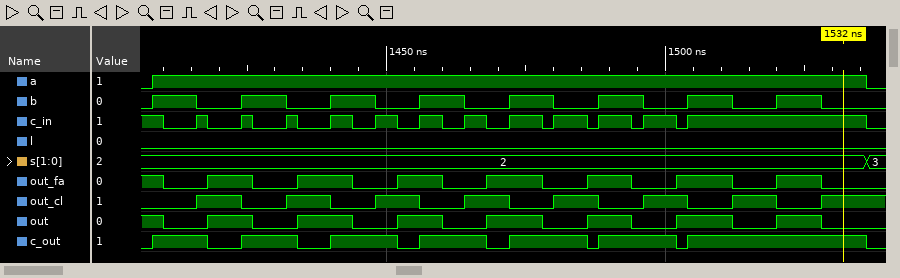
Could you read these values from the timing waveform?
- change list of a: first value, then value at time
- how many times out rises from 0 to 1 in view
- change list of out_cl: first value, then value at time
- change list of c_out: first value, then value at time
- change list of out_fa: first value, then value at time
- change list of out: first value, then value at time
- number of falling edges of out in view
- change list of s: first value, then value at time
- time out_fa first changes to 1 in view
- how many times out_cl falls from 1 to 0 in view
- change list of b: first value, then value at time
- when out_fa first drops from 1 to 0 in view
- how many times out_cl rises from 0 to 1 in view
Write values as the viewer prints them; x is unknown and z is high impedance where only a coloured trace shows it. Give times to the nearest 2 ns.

0, 1 at 1408 ns, 0 at 1536 ns
7
0, 1 at 1416 ns, 0 at 1424 ns, 1 at 1432 ns, 0 at 1440 ns, 1 at 1448 ns, 0 at 1456 ns, 1 at 1464 ns, 0 at 1472 ns, 1 at 1480 ns, 0 at 1488 ns, 1 at 1496 ns, 0 at 1504 ns, 1 at 1512 ns, 0 at 1520 ns, 1 at 1528 ns
0, 1 at 1408 ns, 0 at 1418 ns, 1 at 1424 ns, 0 at 1434 ns, 1 at 1440 ns, 0 at 1452 ns, 1 at 1456 ns, 0 at 1468 ns, 1 at 1472 ns, 0 at 1486 ns, 1 at 1488 ns, 0 at 1502 ns, 1 at 1504 ns, 0 at 1536 ns
1, 0 at 1410 ns, 1 at 1418 ns, 0 at 1426 ns, 1 at 1434 ns, 0 at 1444 ns, 1 at 1452 ns, 0 at 1460 ns, 1 at 1468 ns, 0 at 1478 ns, 1 at 1486 ns, 0 at 1494 ns, 1 at 1502 ns, 0 at 1512 ns, 1 at 1520 ns, 0 at 1528 ns
1, 0 at 1410 ns, 1 at 1418 ns, 0 at 1426 ns, 1 at 1434 ns, 0 at 1444 ns, 1 at 1452 ns, 0 at 1460 ns, 1 at 1468 ns, 0 at 1478 ns, 1 at 1486 ns, 0 at 1494 ns, 1 at 1502 ns, 0 at 1512 ns, 1 at 1520 ns, 0 at 1528 ns
8
2, 3 at 1536 ns
1418 ns
7
0, 1 at 1408 ns, 0 at 1416 ns, 1 at 1424 ns, 0 at 1432 ns, 1 at 1440 ns, 0 at 1448 ns, 1 at 1456 ns, 0 at 1464 ns, 1 at 1472 ns, 0 at 1480 ns, 1 at 1488 ns, 0 at 1496 ns, 1 at 1504 ns, 0 at 1512 ns, 1 at 1520 ns, 0 at 1528 ns
1410 ns
8
